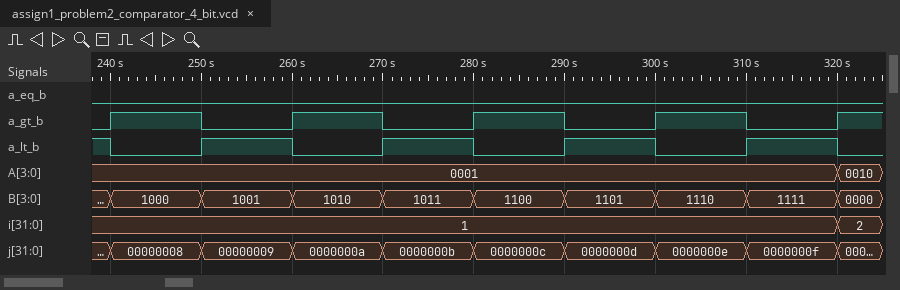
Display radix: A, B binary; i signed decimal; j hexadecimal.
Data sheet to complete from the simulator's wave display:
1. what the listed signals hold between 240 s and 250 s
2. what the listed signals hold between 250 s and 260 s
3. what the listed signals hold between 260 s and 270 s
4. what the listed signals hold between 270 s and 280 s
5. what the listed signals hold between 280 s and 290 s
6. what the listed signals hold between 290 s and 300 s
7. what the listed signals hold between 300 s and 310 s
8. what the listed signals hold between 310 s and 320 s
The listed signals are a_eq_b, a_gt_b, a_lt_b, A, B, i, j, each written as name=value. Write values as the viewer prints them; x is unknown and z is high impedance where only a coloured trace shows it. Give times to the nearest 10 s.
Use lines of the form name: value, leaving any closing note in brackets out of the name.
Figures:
what the listed signals hold between 240 s and 250 s: a_eq_b=0, a_gt_b=1, a_lt_b=0, A=0001, B=1000, i=1, j=00000008
what the listed signals hold between 250 s and 260 s: a_eq_b=0, a_gt_b=0, a_lt_b=1, A=0001, B=1001, i=1, j=00000009
what the listed signals hold between 260 s and 270 s: a_eq_b=0, a_gt_b=1, a_lt_b=0, A=0001, B=1010, i=1, j=0000000a
what the listed signals hold between 270 s and 280 s: a_eq_b=0, a_gt_b=0, a_lt_b=1, A=0001, B=1011, i=1, j=0000000b
what the listed signals hold between 280 s and 290 s: a_eq_b=0, a_gt_b=1, a_lt_b=0, A=0001, B=1100, i=1, j=0000000c
what the listed signals hold between 290 s and 300 s: a_eq_b=0, a_gt_b=0, a_lt_b=1, A=0001, B=1101, i=1, j=0000000d
what the listed signals hold between 300 s and 310 s: a_eq_b=0, a_gt_b=1, a_lt_b=0, A=0001, B=1110, i=1, j=0000000e
what the listed signals hold between 310 s and 320 s: a_eq_b=0, a_gt_b=0, a_lt_b=1, A=0001, B=1111, i=1, j=0000000f
